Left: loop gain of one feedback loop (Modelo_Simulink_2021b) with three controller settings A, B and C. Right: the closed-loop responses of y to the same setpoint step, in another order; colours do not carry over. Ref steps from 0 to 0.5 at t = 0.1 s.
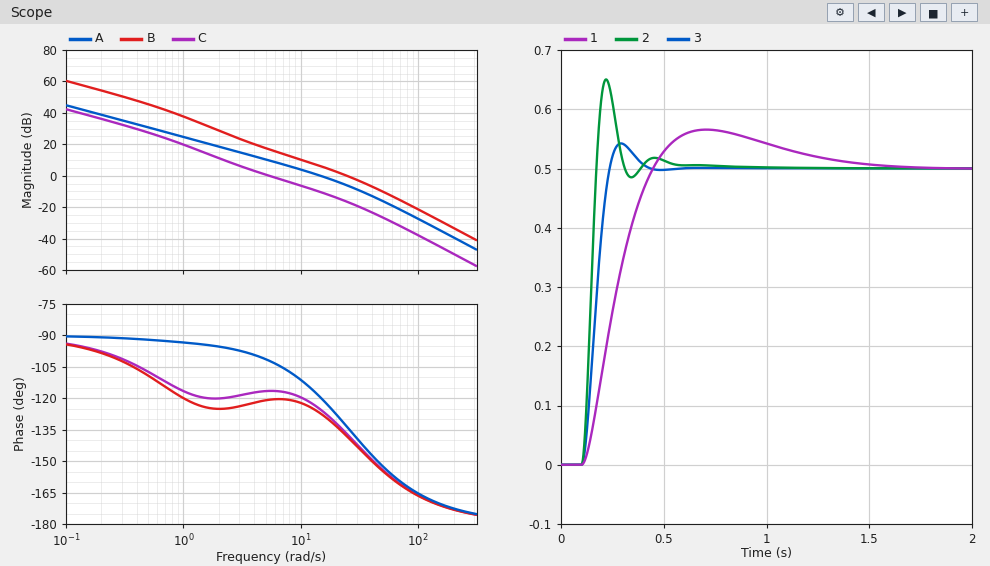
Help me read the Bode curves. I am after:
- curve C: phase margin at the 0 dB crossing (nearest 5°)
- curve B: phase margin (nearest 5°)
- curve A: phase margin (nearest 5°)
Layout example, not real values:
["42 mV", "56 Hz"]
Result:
["65°", "40°", "60°"]
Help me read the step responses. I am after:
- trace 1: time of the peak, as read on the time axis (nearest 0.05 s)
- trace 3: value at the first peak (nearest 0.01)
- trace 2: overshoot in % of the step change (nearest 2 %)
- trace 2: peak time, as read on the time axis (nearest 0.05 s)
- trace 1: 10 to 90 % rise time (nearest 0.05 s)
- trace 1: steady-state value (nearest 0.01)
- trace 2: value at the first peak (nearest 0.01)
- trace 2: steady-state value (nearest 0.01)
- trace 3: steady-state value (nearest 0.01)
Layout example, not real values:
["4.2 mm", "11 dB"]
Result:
["0.70 s", "0.54", "30 %", "0.20 s", "0.25 s", "0.50", "0.65", "0.50", "0.50"]
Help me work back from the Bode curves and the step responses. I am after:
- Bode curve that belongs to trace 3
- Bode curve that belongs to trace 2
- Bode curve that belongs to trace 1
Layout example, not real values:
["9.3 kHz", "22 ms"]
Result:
["A", "B", "C"]
